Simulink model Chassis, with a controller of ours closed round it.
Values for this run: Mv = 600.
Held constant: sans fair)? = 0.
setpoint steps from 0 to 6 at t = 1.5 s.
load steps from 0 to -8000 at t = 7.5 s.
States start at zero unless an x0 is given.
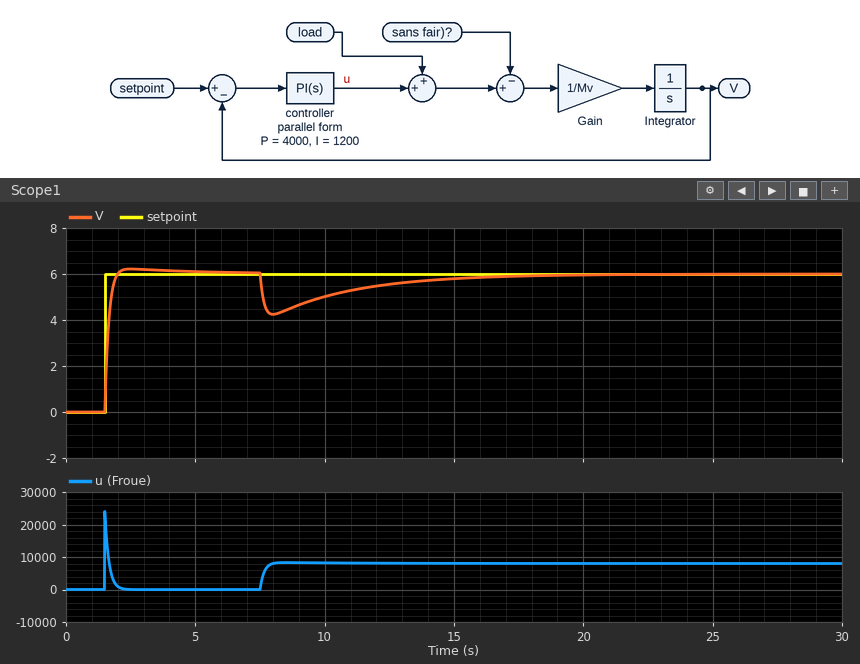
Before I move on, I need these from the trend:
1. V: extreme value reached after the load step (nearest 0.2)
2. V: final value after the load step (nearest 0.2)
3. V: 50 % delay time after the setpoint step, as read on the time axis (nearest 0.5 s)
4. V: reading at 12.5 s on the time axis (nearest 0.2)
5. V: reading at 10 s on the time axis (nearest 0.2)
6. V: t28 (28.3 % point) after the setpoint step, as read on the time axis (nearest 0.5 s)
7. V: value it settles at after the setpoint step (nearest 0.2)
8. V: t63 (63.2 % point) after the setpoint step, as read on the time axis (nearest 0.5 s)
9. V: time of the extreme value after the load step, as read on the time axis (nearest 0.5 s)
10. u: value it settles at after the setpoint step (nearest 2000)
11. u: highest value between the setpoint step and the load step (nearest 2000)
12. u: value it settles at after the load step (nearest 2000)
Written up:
4.2
6.0
1.5 s
5.6
5.0
1.5 s
6.0
1.5 s
8.0 s
0
24000
8000
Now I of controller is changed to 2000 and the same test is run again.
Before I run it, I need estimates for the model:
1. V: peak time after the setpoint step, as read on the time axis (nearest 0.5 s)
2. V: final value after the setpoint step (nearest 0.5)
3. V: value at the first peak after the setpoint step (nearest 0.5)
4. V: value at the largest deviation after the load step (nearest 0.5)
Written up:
2.5 s
6.0
6.5
4.5
